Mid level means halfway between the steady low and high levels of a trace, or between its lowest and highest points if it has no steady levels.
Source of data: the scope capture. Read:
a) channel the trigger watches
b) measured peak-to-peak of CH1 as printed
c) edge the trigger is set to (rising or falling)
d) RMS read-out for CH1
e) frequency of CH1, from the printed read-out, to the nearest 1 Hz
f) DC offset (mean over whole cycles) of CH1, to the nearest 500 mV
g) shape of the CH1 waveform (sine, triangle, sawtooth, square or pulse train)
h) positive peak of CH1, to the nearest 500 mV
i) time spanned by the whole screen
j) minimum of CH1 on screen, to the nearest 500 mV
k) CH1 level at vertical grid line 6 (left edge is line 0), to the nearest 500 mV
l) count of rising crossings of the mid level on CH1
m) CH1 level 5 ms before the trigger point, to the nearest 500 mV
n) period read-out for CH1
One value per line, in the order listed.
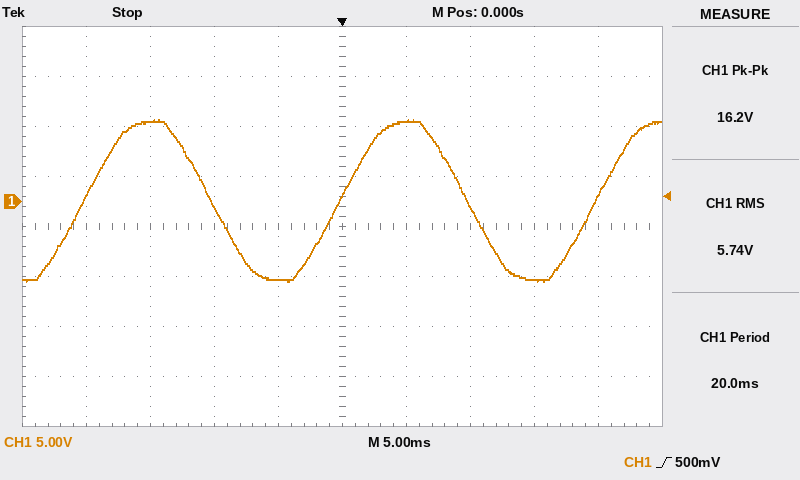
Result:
CH1
16.2 V
rising
5.74 V
50 Hz
0.0 V
sine
8.0 V
50 ms
-8.0 V
8.0 V
3
-8.0 V
20.0 ms
